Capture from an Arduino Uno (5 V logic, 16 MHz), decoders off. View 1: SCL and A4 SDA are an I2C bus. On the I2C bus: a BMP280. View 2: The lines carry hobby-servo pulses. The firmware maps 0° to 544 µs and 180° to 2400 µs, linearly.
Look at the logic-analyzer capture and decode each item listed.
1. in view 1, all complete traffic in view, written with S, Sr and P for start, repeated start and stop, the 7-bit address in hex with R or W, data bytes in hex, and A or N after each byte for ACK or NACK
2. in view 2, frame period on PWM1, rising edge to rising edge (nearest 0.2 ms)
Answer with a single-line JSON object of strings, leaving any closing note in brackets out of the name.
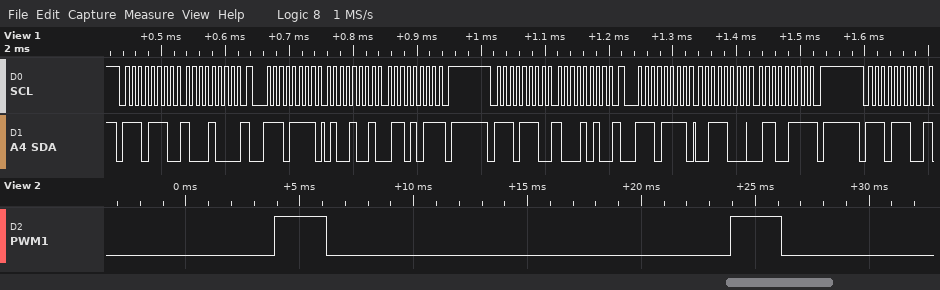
{"in view 1, all complete traffic in view, written with S, Sr and P for start, repeated start and stop, the 7-bit address in hex with R or W, data bytes in hex, and A or N after each byte for ACK or NACK": "S 77W A 88 A Sr 77R A 49 A 6B N P S 77W A 8A A Sr 77R A 38 A 67 N P S 77W A", "in view 2, frame period on PWM1, rising edge to rising edge": "20.0 ms"}
